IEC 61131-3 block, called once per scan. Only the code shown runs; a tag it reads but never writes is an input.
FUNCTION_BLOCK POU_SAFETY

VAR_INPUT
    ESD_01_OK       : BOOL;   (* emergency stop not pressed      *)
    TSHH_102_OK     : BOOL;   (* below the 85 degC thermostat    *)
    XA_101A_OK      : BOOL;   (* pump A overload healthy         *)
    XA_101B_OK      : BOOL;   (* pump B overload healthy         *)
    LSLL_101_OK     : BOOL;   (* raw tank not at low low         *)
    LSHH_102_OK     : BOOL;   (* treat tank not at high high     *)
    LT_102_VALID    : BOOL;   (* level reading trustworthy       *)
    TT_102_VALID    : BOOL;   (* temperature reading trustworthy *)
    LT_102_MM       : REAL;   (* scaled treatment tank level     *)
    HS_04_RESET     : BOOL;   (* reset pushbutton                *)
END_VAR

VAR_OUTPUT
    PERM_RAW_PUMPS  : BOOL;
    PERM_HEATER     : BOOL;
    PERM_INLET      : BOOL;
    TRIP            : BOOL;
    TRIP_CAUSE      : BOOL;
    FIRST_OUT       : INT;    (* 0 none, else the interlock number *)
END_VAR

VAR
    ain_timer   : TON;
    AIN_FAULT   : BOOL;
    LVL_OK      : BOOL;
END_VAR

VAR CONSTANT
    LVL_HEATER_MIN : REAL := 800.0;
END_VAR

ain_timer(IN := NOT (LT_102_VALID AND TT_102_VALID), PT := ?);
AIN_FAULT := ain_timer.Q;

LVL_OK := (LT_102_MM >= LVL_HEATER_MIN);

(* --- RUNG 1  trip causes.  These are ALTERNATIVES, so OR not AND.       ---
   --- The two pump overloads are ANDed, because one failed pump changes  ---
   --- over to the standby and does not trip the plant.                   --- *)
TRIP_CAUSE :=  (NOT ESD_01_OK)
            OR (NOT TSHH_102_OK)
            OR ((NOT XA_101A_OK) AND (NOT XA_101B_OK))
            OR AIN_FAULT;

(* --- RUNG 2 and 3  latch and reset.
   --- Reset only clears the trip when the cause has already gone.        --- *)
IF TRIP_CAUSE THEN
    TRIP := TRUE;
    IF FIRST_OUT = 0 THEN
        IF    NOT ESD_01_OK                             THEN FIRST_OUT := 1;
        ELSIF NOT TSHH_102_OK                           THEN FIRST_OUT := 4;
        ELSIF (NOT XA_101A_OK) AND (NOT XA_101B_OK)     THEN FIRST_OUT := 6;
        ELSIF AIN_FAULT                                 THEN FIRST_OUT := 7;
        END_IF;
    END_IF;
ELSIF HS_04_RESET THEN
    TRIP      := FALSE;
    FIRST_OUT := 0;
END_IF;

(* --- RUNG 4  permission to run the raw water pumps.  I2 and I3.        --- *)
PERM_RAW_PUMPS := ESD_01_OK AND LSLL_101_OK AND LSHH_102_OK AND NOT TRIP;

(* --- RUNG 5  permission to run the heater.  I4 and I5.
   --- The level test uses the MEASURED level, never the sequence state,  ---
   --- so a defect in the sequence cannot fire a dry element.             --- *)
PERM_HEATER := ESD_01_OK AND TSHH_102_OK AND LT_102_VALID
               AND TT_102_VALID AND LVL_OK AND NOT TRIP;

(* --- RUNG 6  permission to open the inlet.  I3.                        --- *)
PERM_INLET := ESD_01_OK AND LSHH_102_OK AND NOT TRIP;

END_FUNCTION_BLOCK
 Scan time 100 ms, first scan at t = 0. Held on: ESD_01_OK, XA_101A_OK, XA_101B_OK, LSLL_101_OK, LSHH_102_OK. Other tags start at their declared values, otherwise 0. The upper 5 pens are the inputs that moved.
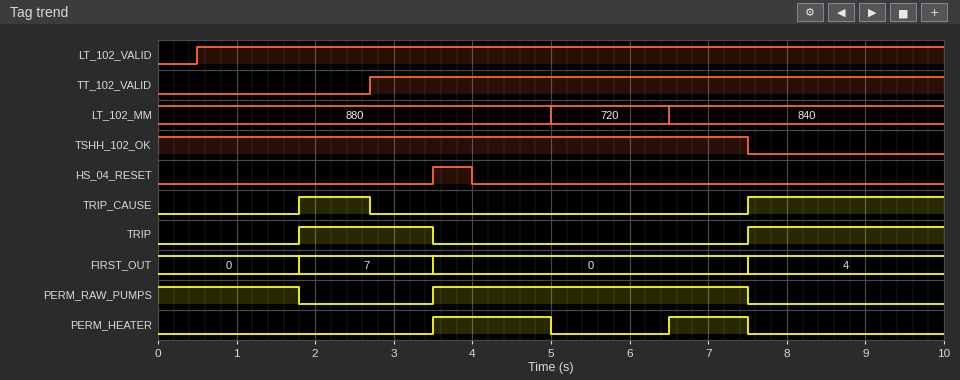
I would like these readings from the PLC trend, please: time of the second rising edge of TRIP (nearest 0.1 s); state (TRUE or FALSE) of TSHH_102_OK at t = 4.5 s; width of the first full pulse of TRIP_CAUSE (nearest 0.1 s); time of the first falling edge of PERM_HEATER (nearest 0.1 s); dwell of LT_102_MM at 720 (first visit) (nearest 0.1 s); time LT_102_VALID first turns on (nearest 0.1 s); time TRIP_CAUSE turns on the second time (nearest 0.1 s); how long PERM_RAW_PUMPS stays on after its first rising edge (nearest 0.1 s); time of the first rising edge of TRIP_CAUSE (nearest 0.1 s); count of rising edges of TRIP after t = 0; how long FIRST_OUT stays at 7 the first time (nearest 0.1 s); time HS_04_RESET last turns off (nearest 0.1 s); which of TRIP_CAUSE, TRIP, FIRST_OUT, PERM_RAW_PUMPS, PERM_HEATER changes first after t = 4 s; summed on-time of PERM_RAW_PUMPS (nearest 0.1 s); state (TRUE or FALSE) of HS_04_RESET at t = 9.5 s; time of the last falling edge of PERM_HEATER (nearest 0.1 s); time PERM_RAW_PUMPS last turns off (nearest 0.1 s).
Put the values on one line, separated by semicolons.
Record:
7.5 s; TRUE; 0.9 s; 5.0 s; 1.5 s; 0.5 s; 7.5 s; 4.0 s; 1.8 s; 2; 1.7 s; 4.0 s; PERM_HEATER; 5.8 s; FALSE; 7.5 s; 7.5 s
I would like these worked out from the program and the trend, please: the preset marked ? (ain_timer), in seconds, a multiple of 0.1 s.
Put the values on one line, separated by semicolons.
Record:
1.8 s
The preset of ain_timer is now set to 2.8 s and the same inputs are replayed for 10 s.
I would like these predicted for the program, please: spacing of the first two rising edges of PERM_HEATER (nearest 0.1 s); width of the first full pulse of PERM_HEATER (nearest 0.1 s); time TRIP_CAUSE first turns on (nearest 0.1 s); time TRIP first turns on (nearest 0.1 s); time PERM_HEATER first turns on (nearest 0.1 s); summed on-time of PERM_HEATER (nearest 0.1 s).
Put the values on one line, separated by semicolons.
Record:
3.8 s; 2.3 s; 7.5 s; 7.5 s; 2.7 s; 3.3 s
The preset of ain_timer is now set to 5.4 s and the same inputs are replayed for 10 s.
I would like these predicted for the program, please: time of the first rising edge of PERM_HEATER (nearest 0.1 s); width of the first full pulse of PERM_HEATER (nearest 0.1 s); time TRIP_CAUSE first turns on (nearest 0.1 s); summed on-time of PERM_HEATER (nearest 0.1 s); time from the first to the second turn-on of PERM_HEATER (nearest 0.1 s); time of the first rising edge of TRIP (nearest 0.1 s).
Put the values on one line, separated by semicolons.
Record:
2.7 s; 2.3 s; 7.5 s; 3.3 s; 3.8 s; 7.5 s
